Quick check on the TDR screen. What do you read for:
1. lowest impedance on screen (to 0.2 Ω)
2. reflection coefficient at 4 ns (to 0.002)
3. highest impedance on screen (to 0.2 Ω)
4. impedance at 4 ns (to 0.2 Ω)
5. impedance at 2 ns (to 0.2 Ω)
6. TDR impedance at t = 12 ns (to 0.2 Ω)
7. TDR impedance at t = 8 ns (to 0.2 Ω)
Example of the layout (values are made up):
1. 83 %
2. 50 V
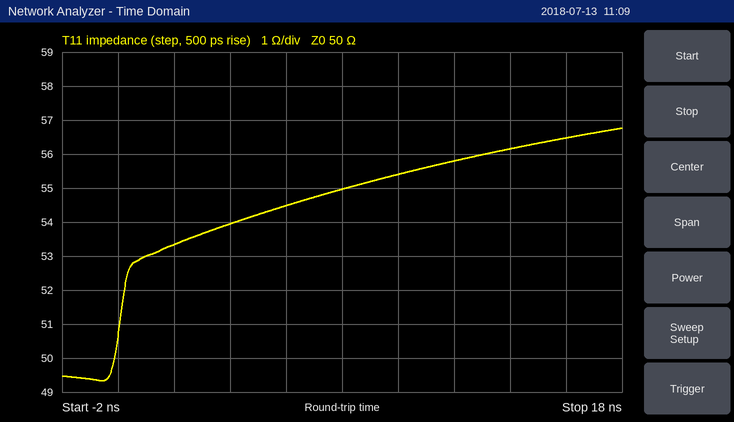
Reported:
1. 49.4 Ω
2. +0.038
3. 56.8 Ω
4. 54.0 Ω
5. 53.4 Ω
6. 55.8 Ω
7. 55.0 Ω
